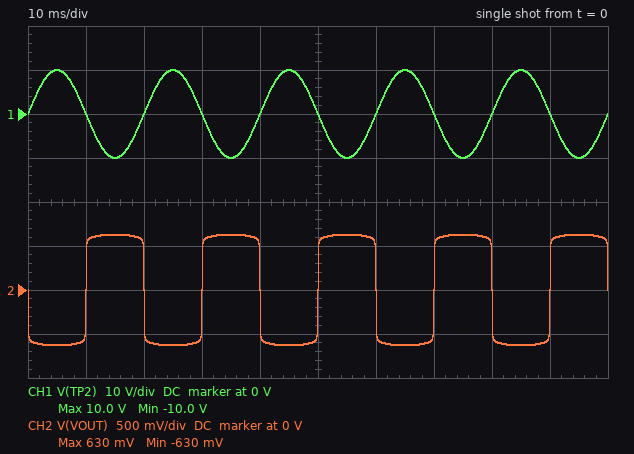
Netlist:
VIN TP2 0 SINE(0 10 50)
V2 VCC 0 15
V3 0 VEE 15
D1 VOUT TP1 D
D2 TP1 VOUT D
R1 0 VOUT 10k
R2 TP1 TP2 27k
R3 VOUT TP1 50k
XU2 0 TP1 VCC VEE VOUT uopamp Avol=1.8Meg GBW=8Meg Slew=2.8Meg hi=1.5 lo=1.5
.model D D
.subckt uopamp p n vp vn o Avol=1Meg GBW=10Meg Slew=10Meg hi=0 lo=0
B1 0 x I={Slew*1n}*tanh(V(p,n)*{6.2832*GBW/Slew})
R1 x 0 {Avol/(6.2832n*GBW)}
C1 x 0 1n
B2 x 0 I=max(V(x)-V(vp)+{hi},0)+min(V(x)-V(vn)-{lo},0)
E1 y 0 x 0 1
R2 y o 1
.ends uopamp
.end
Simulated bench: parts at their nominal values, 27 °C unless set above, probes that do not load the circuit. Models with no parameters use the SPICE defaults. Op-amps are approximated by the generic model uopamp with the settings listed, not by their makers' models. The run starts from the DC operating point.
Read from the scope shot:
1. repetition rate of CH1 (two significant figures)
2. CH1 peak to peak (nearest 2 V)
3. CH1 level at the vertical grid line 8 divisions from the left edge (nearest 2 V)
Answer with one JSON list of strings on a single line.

["50 Hz", "20 V", "0 V"]
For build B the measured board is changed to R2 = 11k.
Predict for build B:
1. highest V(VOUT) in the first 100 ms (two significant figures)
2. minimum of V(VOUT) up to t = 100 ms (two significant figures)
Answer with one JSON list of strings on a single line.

["650 mV", "-650 mV"]
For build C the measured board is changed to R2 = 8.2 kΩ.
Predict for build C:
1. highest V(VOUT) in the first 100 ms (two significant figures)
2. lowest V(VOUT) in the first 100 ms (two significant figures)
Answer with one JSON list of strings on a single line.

["660 mV", "-660 mV"]
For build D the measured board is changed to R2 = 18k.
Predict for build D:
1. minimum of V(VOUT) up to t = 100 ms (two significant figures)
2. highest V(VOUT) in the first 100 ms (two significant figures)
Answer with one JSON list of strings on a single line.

["-640 mV", "640 mV"]
